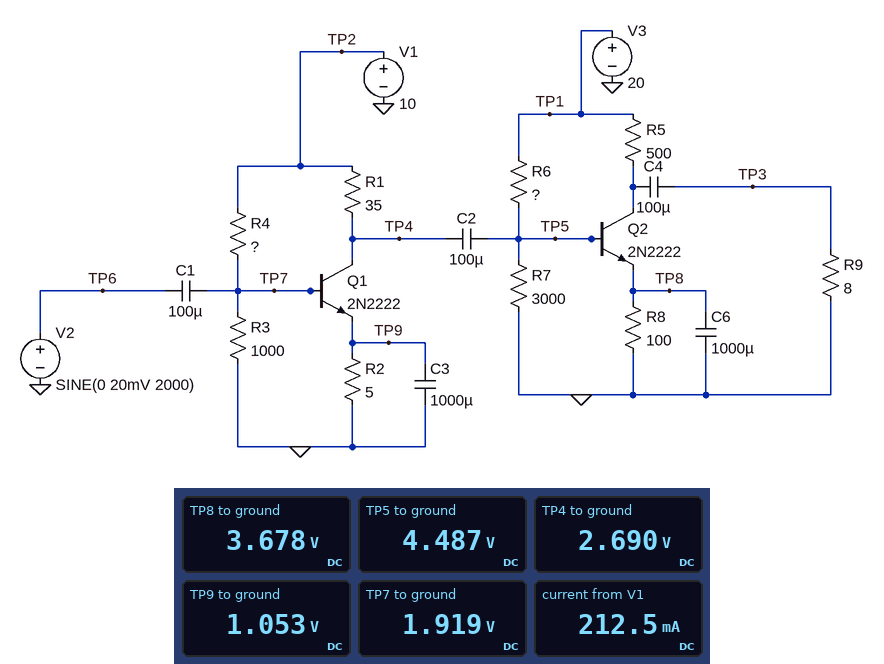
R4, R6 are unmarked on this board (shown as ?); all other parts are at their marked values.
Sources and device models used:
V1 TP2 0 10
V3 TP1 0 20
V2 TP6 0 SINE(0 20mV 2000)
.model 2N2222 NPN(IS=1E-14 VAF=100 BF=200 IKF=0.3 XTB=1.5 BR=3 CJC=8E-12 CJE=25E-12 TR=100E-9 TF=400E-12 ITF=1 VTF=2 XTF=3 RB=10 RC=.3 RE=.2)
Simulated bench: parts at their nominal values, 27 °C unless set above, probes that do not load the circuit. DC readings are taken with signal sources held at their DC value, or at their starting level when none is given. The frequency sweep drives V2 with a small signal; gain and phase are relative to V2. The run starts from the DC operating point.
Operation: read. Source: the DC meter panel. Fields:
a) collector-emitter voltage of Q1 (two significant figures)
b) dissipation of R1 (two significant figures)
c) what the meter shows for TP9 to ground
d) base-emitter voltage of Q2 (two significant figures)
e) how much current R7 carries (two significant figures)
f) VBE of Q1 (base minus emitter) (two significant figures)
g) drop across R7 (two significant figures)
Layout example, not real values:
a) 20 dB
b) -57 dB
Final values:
a) 1.6 V
b) 1.5 W
c) 1.053 V
d) 810 mV
e) 1.5 mA
f) 870 mV
g) 4.5 V
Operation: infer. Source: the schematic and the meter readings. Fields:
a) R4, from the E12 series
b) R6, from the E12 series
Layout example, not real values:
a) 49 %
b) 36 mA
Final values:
a) 2.2 kΩ
b) 2.7 kΩ
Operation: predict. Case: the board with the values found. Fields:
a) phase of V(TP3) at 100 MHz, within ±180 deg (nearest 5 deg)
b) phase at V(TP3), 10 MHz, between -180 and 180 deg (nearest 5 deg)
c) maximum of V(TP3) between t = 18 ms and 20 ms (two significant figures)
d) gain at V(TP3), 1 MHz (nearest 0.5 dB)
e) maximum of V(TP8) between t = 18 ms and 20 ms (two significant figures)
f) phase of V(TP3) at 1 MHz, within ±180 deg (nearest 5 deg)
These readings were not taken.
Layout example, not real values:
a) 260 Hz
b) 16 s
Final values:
a) 85 deg
b) 155 deg
c) 250 mV
d) 8.5 dB
e) 3.7 V
f) -85 deg
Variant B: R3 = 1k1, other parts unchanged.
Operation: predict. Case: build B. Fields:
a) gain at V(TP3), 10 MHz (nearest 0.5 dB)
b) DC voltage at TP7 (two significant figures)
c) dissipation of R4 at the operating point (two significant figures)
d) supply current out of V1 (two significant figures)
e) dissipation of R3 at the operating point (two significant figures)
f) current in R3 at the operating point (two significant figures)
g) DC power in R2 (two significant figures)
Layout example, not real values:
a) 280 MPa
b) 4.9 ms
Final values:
a) -2.0 dB
b) 2.0 V
c) 29 mW
d) 220 mA
e) 3.5 mW
f) 1.8 mA
g) 240 mW
